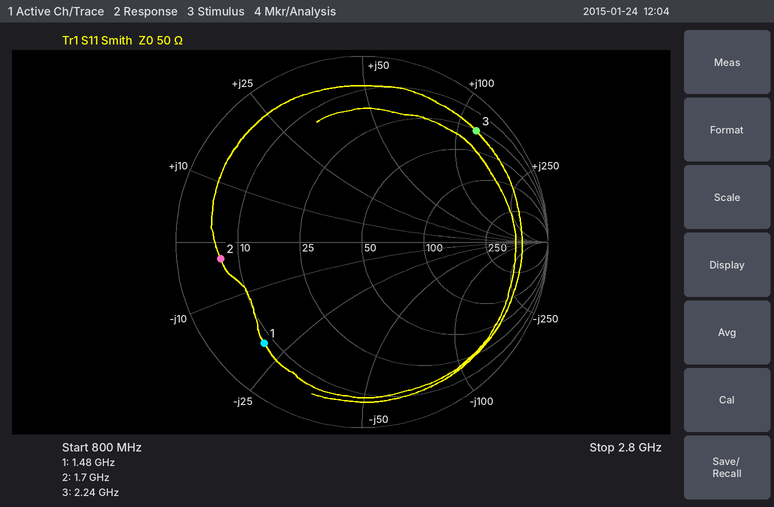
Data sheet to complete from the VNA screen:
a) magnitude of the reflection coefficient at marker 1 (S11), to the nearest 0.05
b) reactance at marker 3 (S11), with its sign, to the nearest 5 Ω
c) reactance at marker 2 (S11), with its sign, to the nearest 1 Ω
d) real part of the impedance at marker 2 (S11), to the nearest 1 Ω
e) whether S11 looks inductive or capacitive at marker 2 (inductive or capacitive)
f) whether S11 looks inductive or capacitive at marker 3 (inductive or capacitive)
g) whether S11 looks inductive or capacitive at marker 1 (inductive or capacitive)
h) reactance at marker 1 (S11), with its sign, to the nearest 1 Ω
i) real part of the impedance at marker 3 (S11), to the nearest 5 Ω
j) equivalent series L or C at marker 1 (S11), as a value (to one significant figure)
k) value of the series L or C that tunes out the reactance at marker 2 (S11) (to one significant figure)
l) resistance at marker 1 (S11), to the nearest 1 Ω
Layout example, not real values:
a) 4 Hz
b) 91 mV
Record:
a) 0.75
b) +120 Ω
c) -3 Ω
d) 7 Ω
e) capacitive
f) inductive
g) capacitive
h) -21 Ω
i) 25 Ω
j) 5 pF
k) 300 pH
l) 8 Ω
